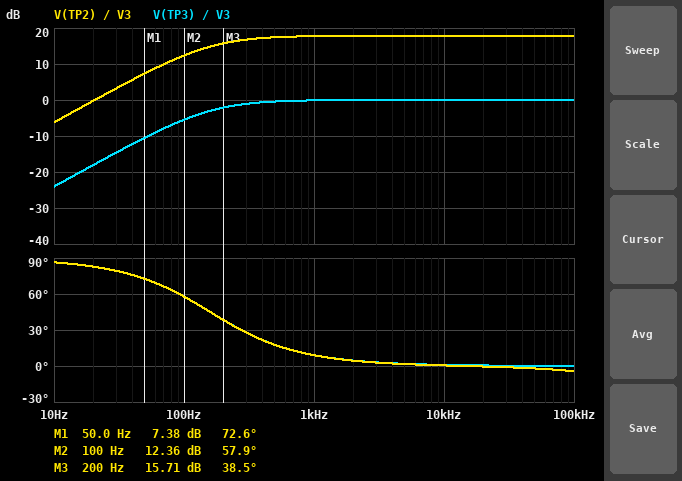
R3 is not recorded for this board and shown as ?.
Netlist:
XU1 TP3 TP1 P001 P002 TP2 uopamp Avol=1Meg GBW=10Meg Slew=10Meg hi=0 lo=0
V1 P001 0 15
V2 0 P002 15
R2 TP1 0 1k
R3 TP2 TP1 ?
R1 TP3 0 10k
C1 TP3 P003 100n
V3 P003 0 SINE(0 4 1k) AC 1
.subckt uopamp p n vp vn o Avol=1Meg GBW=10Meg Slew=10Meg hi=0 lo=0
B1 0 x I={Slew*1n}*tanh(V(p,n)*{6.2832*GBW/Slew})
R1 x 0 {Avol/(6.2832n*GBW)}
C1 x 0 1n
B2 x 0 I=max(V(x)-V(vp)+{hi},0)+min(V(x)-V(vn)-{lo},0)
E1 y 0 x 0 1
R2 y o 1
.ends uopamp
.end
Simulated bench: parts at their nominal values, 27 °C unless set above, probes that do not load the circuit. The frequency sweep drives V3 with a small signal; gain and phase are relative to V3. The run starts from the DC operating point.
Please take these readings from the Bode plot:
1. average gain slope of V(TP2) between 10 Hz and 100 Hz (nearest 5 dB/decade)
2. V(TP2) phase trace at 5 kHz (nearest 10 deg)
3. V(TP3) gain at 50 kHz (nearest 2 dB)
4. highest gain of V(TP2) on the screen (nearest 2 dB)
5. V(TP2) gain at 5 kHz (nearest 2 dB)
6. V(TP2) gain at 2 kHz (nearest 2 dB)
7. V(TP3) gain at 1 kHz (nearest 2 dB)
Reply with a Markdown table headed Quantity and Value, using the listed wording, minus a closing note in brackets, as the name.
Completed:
| Quantity | Value |
|---|---|
| average gain slope of V(TP2) between 10 Hz and 100 Hz | 20 dB/decade |
| V(TP2) phase trace at 5 kHz | 0 deg |
| V(TP3) gain at 50 kHz | 0 dB |
| highest gain of V(TP2) on the screen | 18 dB |
| V(TP2) gain at 5 kHz | 18 dB |
| V(TP2) gain at 2 kHz | 18 dB |
| V(TP3) gain at 1 kHz | 0 dB |
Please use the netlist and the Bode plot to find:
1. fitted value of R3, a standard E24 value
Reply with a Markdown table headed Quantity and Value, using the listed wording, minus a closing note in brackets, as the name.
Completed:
| Quantity | Value |
|---|---|
| fitted value of R3, a standard E24 value | 6.8 kΩ |
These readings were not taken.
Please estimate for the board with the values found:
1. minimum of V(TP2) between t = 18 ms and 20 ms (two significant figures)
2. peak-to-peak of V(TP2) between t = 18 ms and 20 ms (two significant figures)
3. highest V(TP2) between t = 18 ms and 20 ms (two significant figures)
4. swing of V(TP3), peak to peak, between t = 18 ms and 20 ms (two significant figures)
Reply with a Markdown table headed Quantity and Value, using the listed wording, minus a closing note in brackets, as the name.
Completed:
| Quantity | Value |
|---|---|
| minimum of V(TP2) between t = 18 ms and 20 ms | -15 V |
| peak-to-peak of V(TP2) between t = 18 ms and 20 ms | 30 V |
| highest V(TP2) between t = 18 ms and 20 ms | 15 V |
| swing of V(TP3), peak to peak, between t = 18 ms and 20 ms | 7.9 V |
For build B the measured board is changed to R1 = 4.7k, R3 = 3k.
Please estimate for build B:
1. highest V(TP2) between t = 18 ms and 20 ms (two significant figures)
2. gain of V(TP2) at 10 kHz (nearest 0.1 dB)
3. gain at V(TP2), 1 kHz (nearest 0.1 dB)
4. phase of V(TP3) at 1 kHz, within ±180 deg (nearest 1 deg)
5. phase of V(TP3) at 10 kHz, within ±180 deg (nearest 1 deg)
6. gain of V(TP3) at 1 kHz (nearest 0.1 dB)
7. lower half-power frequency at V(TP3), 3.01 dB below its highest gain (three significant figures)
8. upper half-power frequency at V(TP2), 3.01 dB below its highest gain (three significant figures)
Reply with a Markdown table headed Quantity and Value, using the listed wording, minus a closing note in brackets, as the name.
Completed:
| Quantity | Value |
|---|---|
| highest V(TP2) between t = 18 ms and 20 ms | 15 V |
| gain of V(TP2) at 10 kHz | 12.0 dB |
| gain at V(TP2), 1 kHz | 11.6 dB |
| phase of V(TP3) at 1 kHz, within ±180 deg | 19 deg |
| phase of V(TP3) at 10 kHz, within ±180 deg | 2 deg |
| gain of V(TP3) at 1 kHz | -0.5 dB |
| lower half-power frequency at V(TP3), 3.01 dB below its highest gain | 339 Hz |
| upper half-power frequency at V(TP2), 3.01 dB below its highest gain | 2.50 MHz |
